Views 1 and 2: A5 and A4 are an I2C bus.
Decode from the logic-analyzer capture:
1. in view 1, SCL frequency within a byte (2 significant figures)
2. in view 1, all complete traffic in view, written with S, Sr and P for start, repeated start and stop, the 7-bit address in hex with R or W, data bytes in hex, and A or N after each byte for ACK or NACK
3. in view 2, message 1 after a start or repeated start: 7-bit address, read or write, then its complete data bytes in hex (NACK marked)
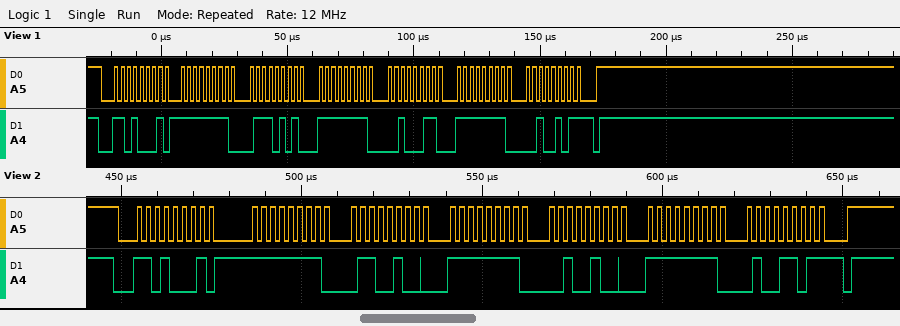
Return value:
400 kHz
S 68R A FF A 75 A FF A 23 A FF A 25 N P
0x68 read: FF 64 FF 24 FF 4D NACK
